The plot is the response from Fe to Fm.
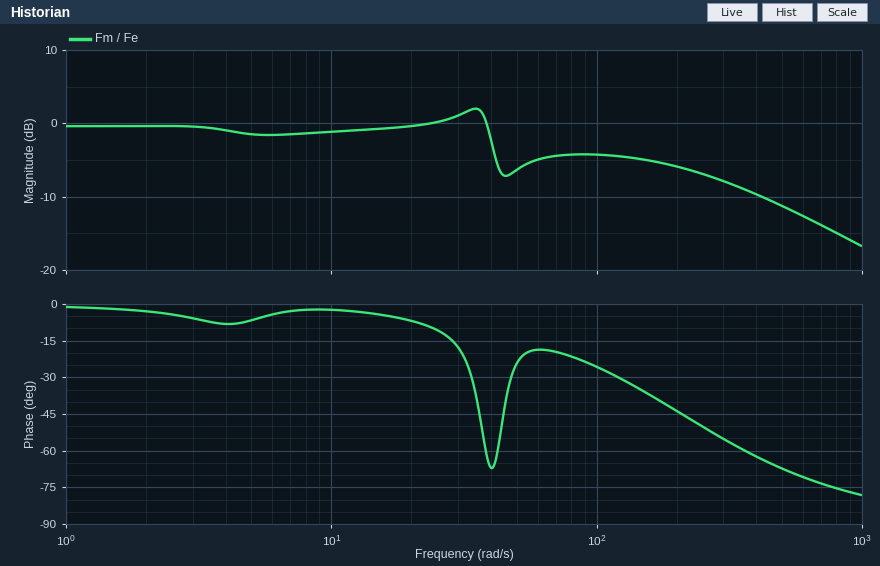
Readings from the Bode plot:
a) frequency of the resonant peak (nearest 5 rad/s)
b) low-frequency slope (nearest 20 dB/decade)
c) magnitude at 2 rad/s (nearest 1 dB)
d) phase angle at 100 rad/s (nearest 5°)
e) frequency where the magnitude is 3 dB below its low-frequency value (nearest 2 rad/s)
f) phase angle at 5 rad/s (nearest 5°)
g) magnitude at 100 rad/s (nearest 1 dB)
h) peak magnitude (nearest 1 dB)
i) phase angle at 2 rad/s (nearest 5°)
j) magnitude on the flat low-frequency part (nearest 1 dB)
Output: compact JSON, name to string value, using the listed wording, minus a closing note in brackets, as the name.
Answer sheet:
{"frequency of the resonant peak": "35 rad/s", "low-frequency slope": "0 dB/decade", "magnitude at 2 rad/s": "0 dB", "phase angle at 100 rad/s": "-25°", "frequency where the magnitude is 3 dB below its low-frequency value": "40 rad/s", "phase angle at 5 rad/s": "-5°", "magnitude at 100 rad/s": "-4 dB", "peak magnitude": "2 dB", "phase angle at 2 rad/s": "-5°", "magnitude on the flat low-frequency part": "0 dB"}
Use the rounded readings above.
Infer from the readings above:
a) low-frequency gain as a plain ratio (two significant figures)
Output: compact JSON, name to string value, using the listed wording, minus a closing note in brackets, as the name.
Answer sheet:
{"low-frequency gain as a plain ratio": "1.0"}
